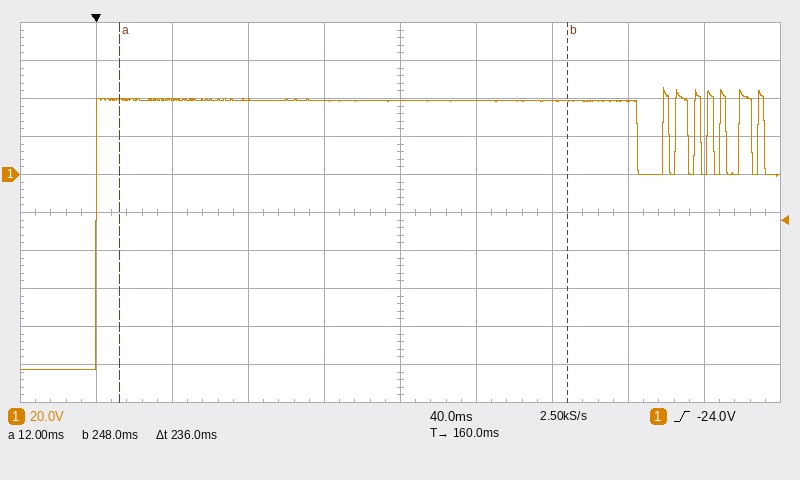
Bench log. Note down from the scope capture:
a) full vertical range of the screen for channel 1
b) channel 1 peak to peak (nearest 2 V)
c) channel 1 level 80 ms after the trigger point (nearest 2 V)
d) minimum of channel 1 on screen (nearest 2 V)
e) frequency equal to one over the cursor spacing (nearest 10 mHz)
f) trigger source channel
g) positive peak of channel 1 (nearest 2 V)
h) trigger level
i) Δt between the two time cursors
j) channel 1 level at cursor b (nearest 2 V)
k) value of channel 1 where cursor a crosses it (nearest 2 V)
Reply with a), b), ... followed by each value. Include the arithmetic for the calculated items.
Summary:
a) 200 V
b) 46 V − (-102 V) = 148 V
c) 40 V
d) -102 V
e) 1 / 236 ms ≈ 4.24 Hz
f) channel 1
g) 46 V
h) -24.0 V
i) 236 ms
j) 38 V
k) 40 V
